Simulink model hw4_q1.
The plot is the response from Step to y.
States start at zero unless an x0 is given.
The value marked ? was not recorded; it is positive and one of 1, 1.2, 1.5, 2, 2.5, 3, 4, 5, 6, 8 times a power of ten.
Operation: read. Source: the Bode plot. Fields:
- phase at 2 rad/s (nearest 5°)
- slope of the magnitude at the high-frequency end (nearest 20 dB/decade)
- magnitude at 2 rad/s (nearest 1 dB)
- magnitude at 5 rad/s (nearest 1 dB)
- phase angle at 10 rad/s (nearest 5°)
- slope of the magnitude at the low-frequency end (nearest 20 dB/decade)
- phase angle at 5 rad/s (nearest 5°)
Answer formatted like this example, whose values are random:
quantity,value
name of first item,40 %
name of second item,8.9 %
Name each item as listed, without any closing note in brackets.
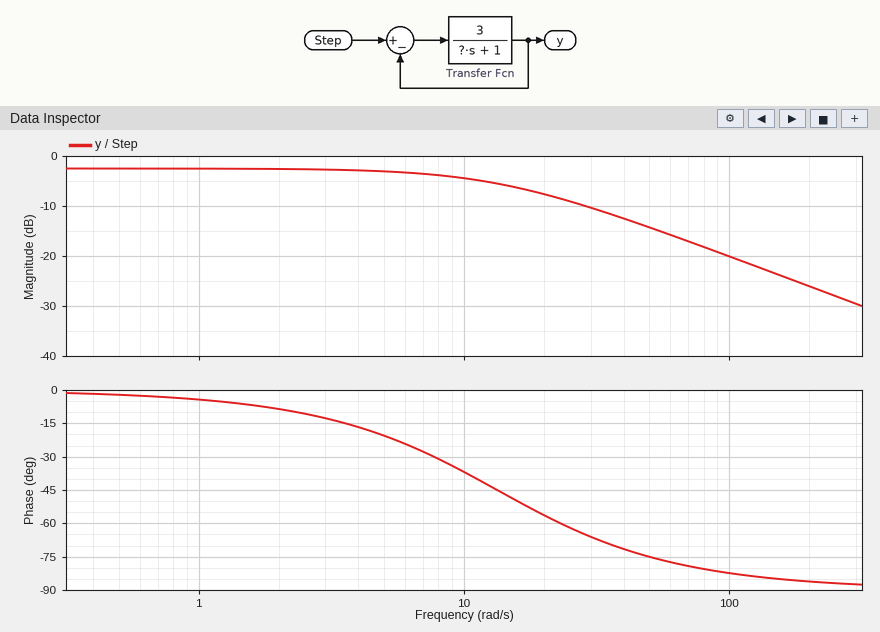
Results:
quantity,value
phase at 2 rad/s,-10°
slope of the magnitude at the high-frequency end,-20 dB/decade
magnitude at 2 rad/s,-3 dB
magnitude at 5 rad/s,-3 dB
phase angle at 10 rad/s,-35°
slope of the magnitude at the low-frequency end,0 dB/decade
phase angle at 5 rad/s,-20°
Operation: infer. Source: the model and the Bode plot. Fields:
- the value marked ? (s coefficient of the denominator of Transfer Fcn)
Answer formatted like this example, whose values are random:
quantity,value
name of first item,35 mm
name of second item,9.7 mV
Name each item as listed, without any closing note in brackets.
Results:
quantity,value
the value marked ?,0.3
